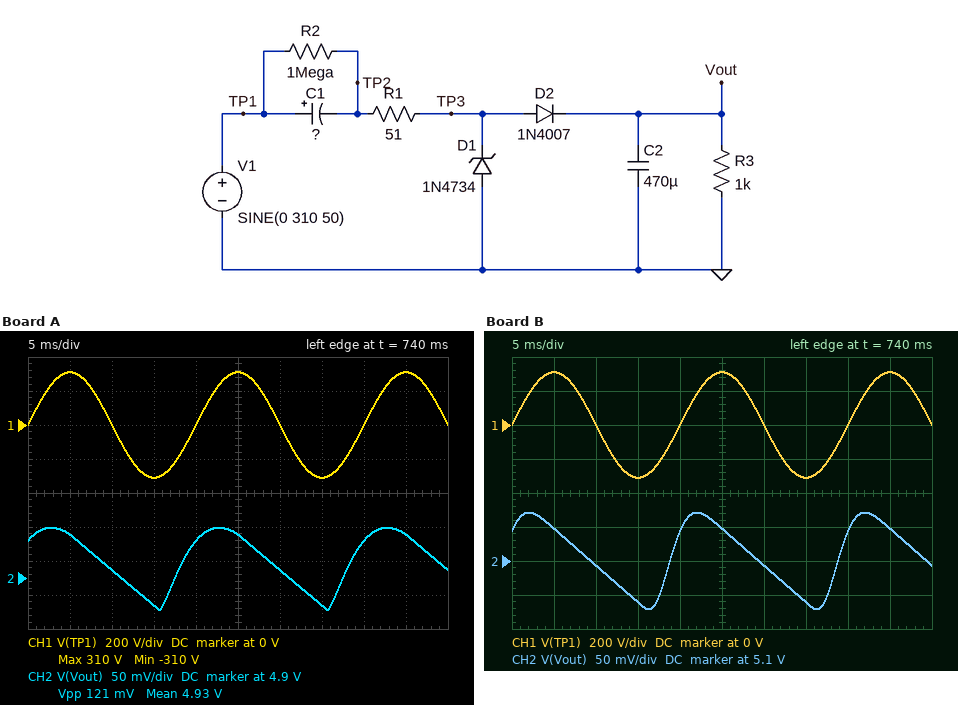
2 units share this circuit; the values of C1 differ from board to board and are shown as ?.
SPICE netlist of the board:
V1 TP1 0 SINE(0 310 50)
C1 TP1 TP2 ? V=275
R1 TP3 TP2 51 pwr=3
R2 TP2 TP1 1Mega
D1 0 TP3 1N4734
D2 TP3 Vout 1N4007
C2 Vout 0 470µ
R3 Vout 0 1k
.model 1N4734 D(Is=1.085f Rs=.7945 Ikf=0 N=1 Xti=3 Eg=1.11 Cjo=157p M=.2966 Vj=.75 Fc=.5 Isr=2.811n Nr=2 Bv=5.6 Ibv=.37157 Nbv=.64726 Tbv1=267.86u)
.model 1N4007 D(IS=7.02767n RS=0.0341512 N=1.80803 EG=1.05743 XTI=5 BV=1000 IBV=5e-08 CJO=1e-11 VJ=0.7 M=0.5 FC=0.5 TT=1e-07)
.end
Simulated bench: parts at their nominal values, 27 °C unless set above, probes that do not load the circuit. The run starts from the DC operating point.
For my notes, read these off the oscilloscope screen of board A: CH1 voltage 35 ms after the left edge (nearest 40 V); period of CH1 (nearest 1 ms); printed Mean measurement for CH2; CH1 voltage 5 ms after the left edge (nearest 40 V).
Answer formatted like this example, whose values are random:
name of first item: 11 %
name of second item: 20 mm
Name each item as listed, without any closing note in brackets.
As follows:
CH1 voltage 35 ms after the left edge: -320 V
period of CH1: 20 ms
printed Mean measurement for CH2: 4.93 V
CH1 voltage 5 ms after the left edge: 320 V
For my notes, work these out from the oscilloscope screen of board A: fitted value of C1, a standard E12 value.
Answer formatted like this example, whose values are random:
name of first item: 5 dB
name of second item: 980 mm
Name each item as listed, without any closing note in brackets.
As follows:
fitted value of C1, a standard E12 value: 820 nF
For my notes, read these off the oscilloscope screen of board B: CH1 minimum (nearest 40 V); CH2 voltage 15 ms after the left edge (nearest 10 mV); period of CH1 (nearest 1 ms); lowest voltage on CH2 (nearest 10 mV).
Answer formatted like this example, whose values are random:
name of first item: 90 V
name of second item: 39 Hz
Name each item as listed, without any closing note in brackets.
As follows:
CH1 minimum: -320 V
CH2 voltage 15 ms after the left edge: 5.04 V
period of CH1: 20 ms
lowest voltage on CH2: 5.03 V
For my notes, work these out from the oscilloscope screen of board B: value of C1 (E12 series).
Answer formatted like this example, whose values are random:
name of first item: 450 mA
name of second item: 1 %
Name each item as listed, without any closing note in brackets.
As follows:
value of C1: 3.3 µF
